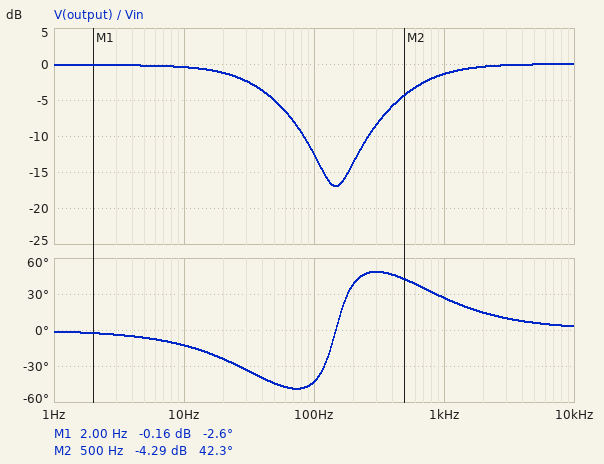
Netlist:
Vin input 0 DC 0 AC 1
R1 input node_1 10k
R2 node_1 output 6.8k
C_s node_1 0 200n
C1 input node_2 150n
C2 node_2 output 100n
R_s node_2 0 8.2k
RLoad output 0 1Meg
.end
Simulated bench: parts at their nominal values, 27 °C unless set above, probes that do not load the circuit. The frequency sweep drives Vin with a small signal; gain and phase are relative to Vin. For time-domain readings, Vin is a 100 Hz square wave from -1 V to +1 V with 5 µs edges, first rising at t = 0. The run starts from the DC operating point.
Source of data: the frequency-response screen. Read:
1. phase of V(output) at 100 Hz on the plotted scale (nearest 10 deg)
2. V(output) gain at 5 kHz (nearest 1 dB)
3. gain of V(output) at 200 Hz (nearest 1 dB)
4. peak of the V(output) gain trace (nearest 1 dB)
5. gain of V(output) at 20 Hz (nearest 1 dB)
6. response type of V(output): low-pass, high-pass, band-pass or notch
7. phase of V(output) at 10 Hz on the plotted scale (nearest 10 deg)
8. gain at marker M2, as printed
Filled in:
-40 deg
0 dB
-14 dB
0 dB
-1 dB
notch
-10 deg
-4.29 dB
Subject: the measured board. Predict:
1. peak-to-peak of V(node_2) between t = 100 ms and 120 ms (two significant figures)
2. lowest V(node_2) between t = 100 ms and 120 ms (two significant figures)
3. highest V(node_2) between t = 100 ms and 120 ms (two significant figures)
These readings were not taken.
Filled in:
3.6 V
-1.8 V
1.8 V
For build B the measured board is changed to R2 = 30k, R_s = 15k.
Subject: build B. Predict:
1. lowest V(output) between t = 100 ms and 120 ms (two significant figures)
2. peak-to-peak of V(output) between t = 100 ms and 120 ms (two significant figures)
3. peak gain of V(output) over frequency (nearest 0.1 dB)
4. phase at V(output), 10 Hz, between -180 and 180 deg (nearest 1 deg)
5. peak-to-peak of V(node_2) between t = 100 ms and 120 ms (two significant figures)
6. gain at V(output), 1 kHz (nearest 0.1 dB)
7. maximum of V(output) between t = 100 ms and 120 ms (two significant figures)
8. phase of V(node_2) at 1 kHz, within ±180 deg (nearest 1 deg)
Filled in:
-1.7 V
3.3 V
0 dB
-20 deg
3.4 V
-0.2 dB
1.7 V
6 deg
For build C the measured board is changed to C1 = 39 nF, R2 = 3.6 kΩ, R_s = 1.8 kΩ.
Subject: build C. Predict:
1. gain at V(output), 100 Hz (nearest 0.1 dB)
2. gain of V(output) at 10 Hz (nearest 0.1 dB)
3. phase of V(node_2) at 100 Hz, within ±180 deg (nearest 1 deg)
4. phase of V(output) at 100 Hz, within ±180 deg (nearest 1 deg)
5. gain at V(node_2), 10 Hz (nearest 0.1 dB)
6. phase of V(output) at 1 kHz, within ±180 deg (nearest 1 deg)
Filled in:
-7.5 dB
-0.3 dB
45 deg
-69 deg
-36.3 dB
87 deg
